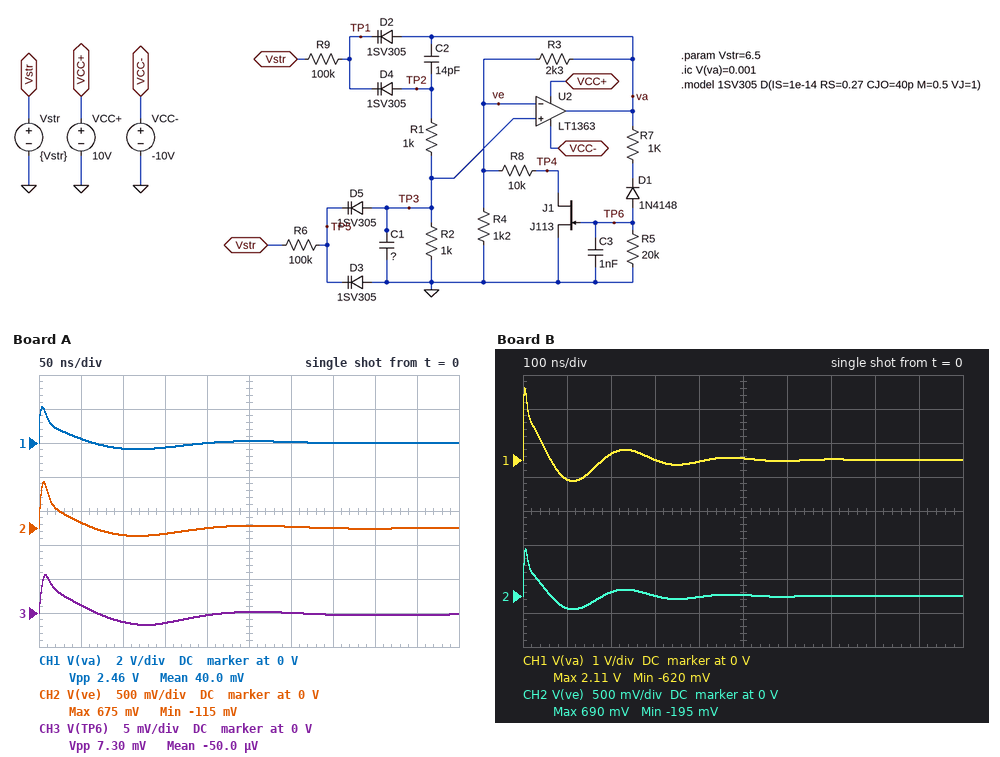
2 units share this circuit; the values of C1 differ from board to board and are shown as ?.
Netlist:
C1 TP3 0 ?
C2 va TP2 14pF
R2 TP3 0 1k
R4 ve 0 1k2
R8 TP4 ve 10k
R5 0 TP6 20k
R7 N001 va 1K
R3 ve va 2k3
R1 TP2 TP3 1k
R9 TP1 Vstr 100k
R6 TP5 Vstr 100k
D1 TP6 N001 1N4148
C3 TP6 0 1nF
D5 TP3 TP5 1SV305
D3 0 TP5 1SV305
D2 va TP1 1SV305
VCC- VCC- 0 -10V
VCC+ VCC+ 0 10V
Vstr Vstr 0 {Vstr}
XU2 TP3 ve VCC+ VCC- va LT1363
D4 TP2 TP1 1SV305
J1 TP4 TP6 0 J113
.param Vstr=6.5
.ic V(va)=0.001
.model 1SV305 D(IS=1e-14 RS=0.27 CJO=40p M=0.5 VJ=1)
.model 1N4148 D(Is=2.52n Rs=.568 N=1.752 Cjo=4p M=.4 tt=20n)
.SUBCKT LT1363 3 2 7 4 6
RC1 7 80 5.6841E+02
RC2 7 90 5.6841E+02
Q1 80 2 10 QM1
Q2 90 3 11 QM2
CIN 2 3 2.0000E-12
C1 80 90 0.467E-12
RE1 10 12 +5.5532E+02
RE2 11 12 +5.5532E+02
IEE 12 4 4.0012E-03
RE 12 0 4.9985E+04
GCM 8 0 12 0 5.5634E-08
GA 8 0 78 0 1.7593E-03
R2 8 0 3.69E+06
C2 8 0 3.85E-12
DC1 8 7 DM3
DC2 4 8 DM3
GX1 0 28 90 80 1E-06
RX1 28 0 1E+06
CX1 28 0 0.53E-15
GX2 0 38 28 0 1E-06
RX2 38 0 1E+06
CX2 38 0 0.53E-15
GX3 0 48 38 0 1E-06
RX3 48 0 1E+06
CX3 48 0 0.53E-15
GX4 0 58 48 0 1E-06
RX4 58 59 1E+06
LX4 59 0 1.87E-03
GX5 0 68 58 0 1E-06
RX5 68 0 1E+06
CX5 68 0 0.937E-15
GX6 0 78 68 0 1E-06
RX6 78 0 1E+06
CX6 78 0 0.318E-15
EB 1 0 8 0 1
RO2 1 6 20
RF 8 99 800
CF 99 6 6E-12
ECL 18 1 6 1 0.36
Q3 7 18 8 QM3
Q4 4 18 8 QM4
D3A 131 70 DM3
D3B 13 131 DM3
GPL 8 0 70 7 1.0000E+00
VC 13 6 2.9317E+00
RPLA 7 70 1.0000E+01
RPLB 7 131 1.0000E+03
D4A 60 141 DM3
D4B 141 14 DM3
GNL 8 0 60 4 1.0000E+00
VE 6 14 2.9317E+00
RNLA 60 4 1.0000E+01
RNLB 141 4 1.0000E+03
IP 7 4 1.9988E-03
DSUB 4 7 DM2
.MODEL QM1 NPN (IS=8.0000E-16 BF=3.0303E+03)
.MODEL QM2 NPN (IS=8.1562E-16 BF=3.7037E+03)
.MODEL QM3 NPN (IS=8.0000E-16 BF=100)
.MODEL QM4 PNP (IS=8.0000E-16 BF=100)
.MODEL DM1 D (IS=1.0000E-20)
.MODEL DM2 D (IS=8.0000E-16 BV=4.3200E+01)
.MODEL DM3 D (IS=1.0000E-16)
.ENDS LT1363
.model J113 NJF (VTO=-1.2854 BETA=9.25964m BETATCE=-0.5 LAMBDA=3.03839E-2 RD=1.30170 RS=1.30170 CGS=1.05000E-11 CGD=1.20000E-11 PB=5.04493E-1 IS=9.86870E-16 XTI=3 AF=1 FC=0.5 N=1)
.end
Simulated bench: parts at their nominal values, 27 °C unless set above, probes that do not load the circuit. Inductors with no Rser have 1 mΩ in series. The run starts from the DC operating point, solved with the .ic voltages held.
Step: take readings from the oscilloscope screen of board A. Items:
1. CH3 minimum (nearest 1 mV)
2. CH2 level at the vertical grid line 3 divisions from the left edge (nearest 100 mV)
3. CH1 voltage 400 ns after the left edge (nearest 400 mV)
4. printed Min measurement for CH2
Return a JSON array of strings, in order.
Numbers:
["-2 mV", "-100 mV", "0 V", "-115 mV"]
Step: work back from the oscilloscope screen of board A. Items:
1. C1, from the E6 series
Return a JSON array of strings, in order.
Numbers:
["47 pF"]
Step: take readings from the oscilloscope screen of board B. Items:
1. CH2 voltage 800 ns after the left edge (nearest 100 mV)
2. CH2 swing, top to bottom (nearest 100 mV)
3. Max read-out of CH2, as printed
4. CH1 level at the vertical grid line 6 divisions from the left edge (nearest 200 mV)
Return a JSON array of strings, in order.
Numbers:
["0 V", "900 mV", "690 mV", "0 V"]
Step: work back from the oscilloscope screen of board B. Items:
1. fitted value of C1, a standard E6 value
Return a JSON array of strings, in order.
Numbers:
["33 pF"]
